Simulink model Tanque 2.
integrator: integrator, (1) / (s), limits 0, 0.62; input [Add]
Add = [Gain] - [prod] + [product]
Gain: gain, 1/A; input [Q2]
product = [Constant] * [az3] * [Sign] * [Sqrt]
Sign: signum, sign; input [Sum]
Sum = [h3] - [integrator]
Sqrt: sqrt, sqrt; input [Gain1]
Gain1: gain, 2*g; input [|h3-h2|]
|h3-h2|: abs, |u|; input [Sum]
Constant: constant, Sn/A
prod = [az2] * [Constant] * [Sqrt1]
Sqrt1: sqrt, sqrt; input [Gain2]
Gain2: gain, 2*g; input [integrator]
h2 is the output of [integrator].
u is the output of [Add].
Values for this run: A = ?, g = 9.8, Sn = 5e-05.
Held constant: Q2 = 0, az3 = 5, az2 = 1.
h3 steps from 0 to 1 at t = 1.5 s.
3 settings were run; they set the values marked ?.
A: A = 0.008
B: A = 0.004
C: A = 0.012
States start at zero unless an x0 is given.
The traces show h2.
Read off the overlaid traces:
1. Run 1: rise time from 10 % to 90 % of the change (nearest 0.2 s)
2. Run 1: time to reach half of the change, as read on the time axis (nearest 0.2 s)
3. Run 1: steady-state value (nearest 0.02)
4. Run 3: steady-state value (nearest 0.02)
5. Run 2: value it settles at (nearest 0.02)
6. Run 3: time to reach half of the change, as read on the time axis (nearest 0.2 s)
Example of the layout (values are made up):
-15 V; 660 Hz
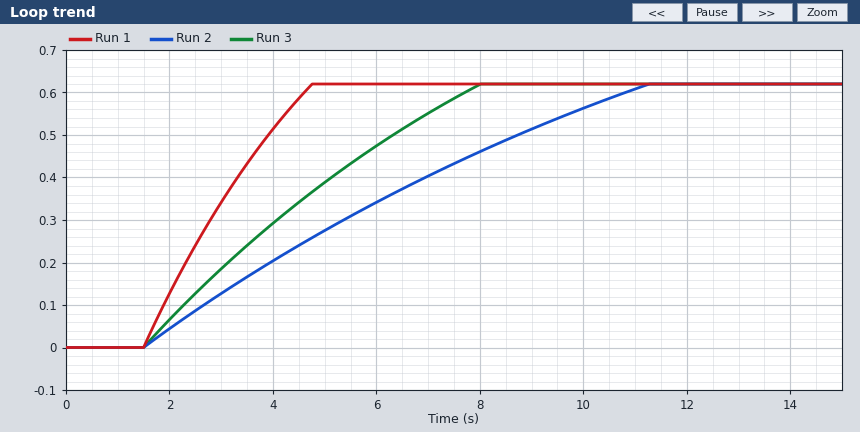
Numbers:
2.6 s; 2.8 s; 0.62; 0.62; 0.62; 4.2 s
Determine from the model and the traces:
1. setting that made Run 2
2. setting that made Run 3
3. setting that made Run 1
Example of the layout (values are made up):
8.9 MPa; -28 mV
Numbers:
C; A; B
